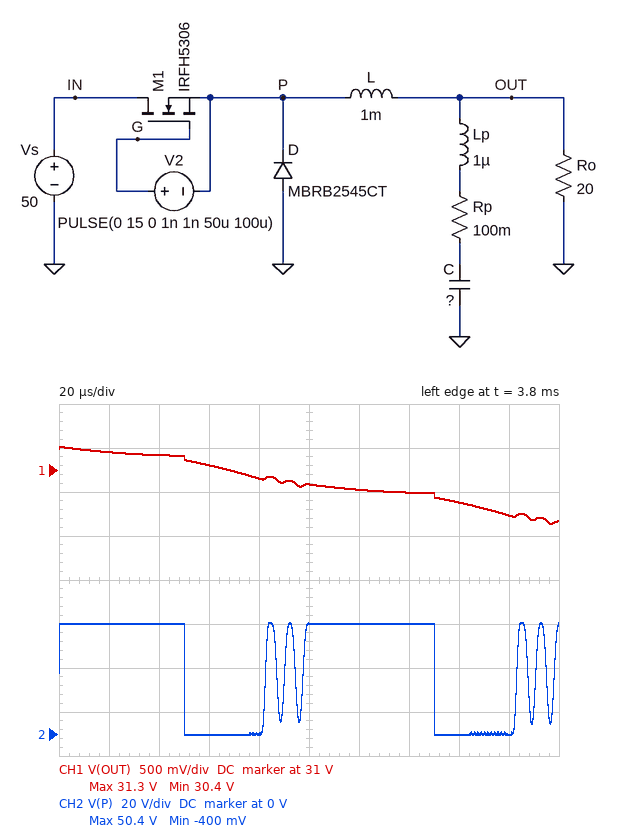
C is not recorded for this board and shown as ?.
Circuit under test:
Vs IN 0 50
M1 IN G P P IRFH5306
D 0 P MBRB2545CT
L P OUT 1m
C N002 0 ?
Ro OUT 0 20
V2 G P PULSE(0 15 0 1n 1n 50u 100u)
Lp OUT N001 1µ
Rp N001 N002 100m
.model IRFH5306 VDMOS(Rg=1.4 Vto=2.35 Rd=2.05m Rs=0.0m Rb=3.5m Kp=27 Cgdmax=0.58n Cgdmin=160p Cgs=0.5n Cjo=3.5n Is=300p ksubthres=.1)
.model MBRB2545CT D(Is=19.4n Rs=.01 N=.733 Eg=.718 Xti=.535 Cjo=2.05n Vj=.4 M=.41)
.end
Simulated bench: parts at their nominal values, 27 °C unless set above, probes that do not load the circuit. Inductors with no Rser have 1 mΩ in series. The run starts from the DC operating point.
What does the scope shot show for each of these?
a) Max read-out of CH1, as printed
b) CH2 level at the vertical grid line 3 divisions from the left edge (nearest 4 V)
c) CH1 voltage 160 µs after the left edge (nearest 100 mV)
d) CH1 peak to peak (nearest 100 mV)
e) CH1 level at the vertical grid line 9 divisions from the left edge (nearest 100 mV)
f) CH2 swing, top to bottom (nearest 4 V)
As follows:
31.3 V
0 V
30.6 V
900 mV
30.5 V
52 V
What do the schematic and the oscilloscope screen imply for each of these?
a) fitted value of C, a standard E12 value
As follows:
270 µF
